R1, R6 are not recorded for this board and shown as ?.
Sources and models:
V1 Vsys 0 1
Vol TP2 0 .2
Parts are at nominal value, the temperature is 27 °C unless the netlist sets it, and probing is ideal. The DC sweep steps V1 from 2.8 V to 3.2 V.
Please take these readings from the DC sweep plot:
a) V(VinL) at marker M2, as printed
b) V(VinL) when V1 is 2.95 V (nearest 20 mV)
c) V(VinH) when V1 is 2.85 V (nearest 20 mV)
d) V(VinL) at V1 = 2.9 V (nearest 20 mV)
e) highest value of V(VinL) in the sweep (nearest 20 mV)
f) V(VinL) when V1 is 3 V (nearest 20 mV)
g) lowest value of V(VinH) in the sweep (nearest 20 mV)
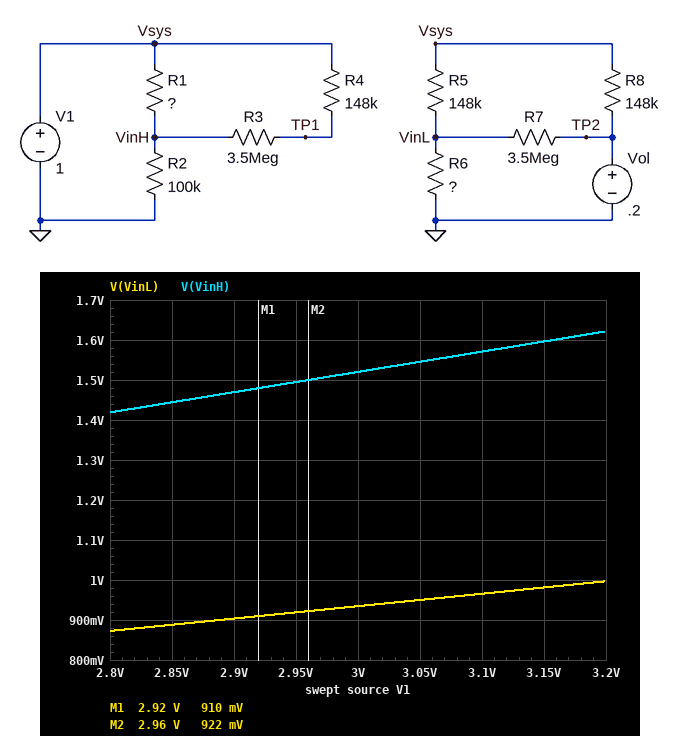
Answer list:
922 mV
920 mV
1.44 V
900 mV
1.00 V
940 mV
1.42 V
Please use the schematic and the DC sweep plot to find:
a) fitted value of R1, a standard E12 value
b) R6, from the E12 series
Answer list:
100 kΩ
68 kΩ
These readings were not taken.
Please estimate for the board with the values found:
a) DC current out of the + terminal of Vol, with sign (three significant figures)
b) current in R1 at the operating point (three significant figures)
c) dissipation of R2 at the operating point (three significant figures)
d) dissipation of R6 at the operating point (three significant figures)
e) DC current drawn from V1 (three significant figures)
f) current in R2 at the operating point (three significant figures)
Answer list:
-5.44 µA
4.93 µA
2.57 µW
1.44 µW
15.1 µA
5.07 µA
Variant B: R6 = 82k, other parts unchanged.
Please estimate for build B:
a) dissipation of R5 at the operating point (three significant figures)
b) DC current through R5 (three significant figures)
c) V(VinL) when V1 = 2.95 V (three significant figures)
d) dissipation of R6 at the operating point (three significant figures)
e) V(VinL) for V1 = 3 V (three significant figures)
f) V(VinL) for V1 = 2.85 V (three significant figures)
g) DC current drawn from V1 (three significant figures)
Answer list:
2.82 µW
4.36 µA
1.04 V
1.53 µW
1.06 V
1.00 V
14.8 µA
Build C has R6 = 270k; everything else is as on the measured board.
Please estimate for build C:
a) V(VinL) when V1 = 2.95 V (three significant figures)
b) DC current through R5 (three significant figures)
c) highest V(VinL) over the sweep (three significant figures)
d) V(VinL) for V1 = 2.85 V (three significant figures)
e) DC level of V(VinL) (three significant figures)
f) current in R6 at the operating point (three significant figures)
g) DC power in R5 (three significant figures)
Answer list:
1.86 V
2.47 µA
2.02 V
1.80 V
634 mV
2.35 µA
905 nW
